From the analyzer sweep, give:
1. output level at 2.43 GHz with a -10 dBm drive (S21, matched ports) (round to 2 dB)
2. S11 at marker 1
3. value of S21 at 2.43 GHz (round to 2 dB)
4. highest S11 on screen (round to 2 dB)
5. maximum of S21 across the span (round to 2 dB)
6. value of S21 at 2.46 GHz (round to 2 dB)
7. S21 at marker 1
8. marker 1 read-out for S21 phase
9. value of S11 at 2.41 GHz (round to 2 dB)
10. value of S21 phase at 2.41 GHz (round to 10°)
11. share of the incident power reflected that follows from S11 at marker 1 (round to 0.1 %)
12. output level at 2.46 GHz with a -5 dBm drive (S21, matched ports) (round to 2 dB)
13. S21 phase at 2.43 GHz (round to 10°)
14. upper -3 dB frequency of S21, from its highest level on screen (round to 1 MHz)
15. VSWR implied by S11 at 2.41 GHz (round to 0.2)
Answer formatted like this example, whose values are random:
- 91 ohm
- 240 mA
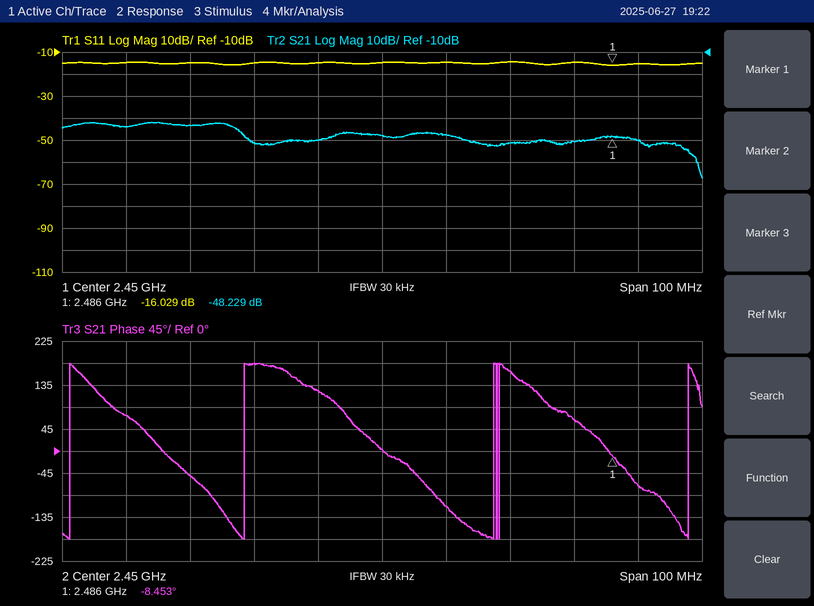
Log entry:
- -62 dBm
- -16.029 dB
- -52 dB
- -14 dB
- -42 dB
- -48 dB
- -48.229 dB
- -8.453°
- -14 dB
- 70°
- 2.5 %
- -52 dBm
- 180°
- 2.427 GHz
- 1.4
